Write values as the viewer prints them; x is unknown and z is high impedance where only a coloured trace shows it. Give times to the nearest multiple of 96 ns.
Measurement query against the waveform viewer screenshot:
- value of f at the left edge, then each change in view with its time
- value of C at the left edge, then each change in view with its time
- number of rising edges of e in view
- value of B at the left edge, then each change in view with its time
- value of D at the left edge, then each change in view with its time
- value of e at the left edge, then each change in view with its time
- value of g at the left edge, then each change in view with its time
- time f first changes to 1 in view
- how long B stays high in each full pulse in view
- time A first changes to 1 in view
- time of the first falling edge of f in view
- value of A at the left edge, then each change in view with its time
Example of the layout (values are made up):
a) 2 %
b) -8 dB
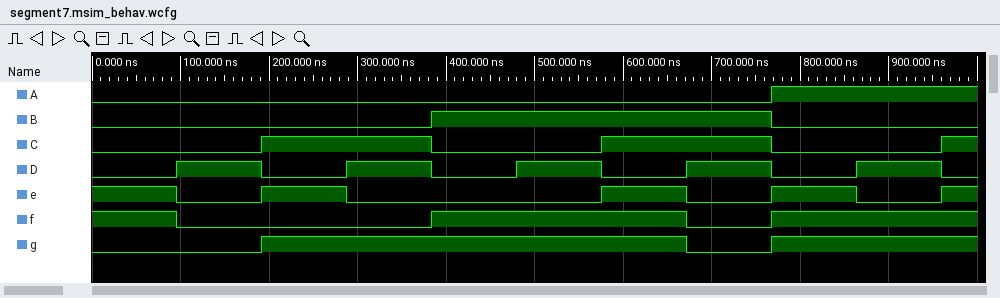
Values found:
a) 1, 0 at 96 ns, 1 at 384 ns, 0 at 672 ns, 1 at 768 ns
b) 0, 1 at 192 ns, 0 at 384 ns, 1 at 576 ns, 0 at 768 ns, 1 at 960 ns
c) 4
d) 0, 1 at 384 ns, 0 at 768 ns
e) 0, 1 at 96 ns, 0 at 192 ns, 1 at 288 ns, 0 at 384 ns, 1 at 480 ns, 0 at 576 ns, 1 at 672 ns, 0 at 768 ns, 1 at 864 ns, 0 at 960 ns
f) 1, 0 at 96 ns, 1 at 192 ns, 0 at 288 ns, 1 at 576 ns, 0 at 672 ns, 1 at 768 ns, 0 at 864 ns, 1 at 960 ns
g) 0, 1 at 192 ns, 0 at 672 ns, 1 at 768 ns
h) 384 ns
i) 384 ns
j) 768 ns
k) 96 ns
l) 0, 1 at 768 ns
